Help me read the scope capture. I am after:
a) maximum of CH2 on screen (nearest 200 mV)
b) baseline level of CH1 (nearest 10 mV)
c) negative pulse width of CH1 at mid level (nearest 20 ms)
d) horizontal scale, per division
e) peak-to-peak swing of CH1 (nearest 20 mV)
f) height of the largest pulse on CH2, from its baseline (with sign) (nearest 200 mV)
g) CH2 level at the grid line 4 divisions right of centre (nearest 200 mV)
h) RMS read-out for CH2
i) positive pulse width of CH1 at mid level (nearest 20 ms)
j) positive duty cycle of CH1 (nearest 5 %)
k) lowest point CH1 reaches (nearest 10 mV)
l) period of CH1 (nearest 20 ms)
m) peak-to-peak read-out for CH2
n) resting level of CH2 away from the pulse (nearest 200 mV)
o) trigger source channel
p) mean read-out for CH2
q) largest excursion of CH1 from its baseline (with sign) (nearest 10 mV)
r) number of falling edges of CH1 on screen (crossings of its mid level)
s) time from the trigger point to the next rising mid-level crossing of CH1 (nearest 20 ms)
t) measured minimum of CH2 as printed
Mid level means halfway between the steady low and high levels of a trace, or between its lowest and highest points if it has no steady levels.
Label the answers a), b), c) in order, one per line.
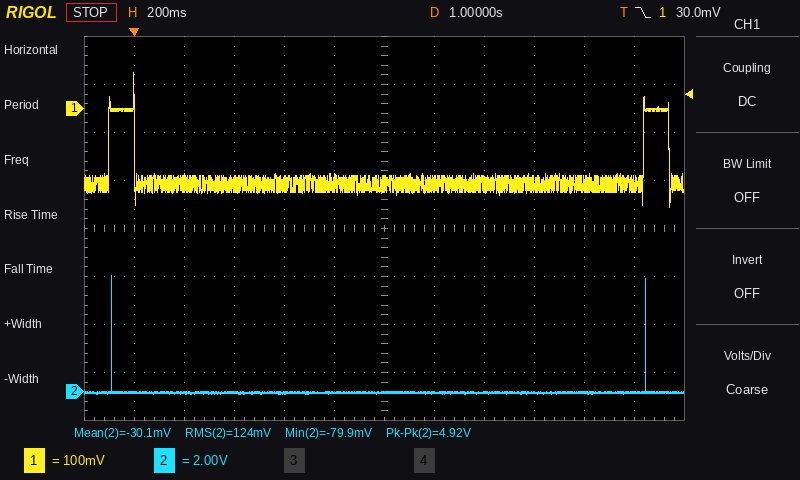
a) 4.8 V
b) -160 mV
c) 2.04 s
d) 200 ms
e) 280 mV
f) +4.8 V
g) 0.0 V
h) 124 mV
i) 100 ms
j) 5 %
k) -200 mV
l) 2.14 s
m) 4.92 V
n) 0.0 V
o) CH1
p) -30.1 mV
q) +230 mV
r) 2
s) 2.04 s
t) -79.9 mV
